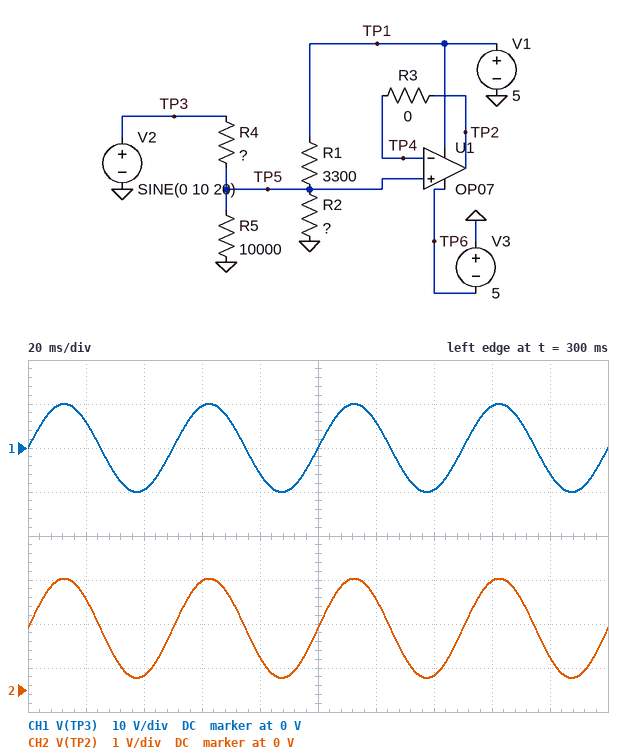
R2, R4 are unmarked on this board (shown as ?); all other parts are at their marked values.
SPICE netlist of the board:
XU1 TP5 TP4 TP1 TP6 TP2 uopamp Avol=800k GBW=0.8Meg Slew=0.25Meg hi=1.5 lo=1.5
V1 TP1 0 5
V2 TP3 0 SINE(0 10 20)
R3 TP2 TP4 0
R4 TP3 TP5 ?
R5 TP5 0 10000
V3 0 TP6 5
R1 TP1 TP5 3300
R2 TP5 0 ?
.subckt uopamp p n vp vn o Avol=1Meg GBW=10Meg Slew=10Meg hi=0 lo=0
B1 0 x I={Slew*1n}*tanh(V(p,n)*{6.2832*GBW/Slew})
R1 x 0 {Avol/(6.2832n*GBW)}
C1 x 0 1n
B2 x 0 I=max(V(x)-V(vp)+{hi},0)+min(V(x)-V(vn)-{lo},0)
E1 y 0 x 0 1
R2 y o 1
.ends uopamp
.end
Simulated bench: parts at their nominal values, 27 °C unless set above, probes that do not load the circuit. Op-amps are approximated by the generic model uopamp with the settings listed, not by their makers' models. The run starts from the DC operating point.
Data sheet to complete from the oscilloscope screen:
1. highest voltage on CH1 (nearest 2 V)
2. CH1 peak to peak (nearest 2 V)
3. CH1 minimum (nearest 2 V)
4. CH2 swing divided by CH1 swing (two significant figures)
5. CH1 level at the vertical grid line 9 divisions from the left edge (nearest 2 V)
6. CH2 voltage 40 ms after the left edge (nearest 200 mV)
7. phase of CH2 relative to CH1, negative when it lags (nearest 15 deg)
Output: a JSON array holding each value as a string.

["10 V", "20 V", "-10 V", "0.11", "-6 V", "400 mV", "0 deg"]
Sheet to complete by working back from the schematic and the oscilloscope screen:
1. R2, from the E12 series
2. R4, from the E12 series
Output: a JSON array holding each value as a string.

["1.8 kΩ", "8.2 kΩ"]
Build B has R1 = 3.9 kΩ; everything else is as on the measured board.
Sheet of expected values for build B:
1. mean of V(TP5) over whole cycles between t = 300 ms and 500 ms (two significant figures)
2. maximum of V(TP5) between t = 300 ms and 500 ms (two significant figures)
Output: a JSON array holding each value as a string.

["1.2 V", "2.4 V"]
